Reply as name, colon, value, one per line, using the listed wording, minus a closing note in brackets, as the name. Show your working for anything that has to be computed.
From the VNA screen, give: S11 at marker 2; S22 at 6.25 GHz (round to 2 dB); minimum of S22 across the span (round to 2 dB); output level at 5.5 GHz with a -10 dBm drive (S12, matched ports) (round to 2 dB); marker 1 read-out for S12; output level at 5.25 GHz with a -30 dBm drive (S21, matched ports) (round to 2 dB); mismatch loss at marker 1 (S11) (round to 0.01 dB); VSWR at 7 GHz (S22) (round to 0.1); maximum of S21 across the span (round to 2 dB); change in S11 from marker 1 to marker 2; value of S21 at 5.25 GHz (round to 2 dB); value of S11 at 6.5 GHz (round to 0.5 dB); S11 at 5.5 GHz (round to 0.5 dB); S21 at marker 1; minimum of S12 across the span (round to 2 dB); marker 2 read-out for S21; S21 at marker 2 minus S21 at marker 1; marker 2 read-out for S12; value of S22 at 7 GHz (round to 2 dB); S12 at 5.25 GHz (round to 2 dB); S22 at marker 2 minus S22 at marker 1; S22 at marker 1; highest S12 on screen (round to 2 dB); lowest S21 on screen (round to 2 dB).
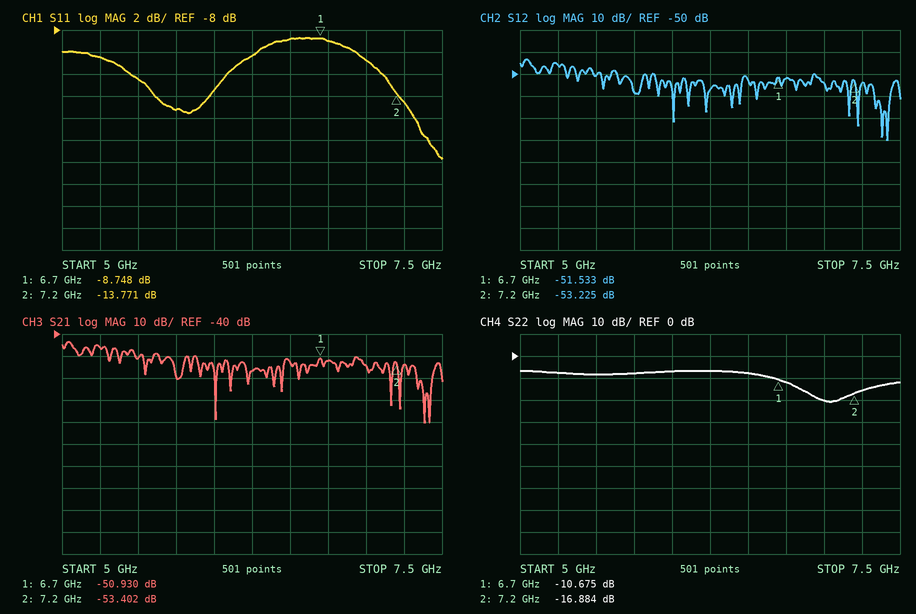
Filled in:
S11 at marker 2: -13.771 dB
S22 at 6.25 GHz: -6 dB
minimum of S22 across the span: -20 dB
output level at 5.5 GHz with a -10 dBm drive (S12, matched ports): -10 dBm + (-50 dB) = -60 dBm
marker 1 read-out for S12: -51.533 dB
output level at 5.25 GHz with a -30 dBm drive (S21, matched ports): -30 dBm + (-46 dB) = -76 dBm
mismatch loss at marker 1 (S11): −10 log10(1 − 10^(-8.748/10)) ≈ 0.62 dB
VSWR at 7 GHz (S22): |Γ| = 10^(-20/20) = 0.1000; VSWR = (1 + 0.1000)/(1 − 0.1000) ≈ 1.2
maximum of S21 across the span: -44 dB
change in S11 from marker 1 to marker 2: -13.771 − (-8.748) = -5.023 dB
value of S21 at 5.25 GHz: -46 dB
value of S11 at 6.5 GHz: -9.0 dB
S11 at 5.5 GHz: -12.5 dB
S21 at marker 1: -50.930 dB
minimum of S12 across the span: -80 dB
marker 2 read-out for S21: -53.402 dB
S21 at marker 2 minus S21 at marker 1: -53.402 − (-50.93) = -2.472 dB
marker 2 read-out for S12: -53.225 dB
value of S22 at 7 GHz: -20 dB
S12 at 5.25 GHz: -46 dB
S22 at marker 2 minus S22 at marker 1: -16.884 − (-10.675) = -6.209 dB
S22 at marker 1: -10.675 dB
highest S12 on screen: -44 dB
lowest S21 on screen: -80 dB
